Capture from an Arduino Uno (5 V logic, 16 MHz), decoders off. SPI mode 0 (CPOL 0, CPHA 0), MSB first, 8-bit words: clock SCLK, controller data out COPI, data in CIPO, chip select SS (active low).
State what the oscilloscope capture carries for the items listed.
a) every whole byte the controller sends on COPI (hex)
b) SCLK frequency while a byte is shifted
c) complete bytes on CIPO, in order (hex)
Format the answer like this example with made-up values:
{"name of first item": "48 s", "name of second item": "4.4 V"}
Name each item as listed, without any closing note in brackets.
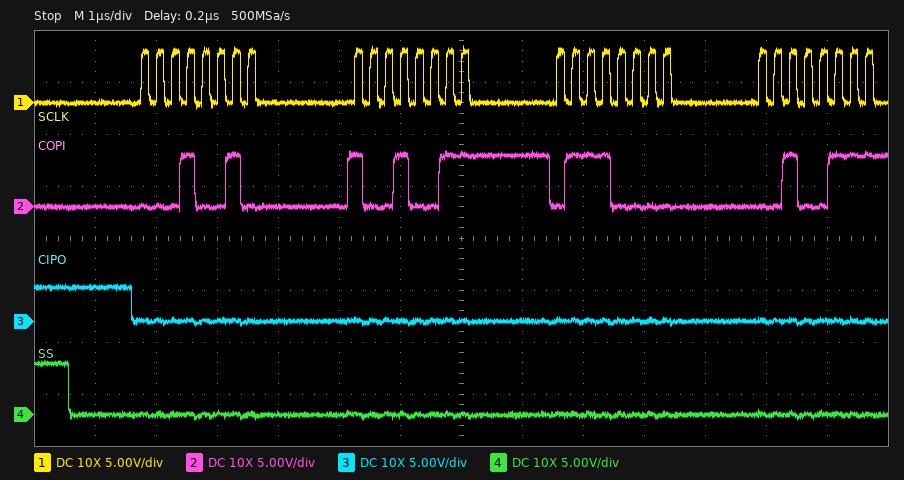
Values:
{"every whole byte the controller sends on COPI": "12 93 70 27", "SCLK frequency while a byte is shifted": "4 MHz", "complete bytes on CIPO, in order": "00 00 00 00"}
